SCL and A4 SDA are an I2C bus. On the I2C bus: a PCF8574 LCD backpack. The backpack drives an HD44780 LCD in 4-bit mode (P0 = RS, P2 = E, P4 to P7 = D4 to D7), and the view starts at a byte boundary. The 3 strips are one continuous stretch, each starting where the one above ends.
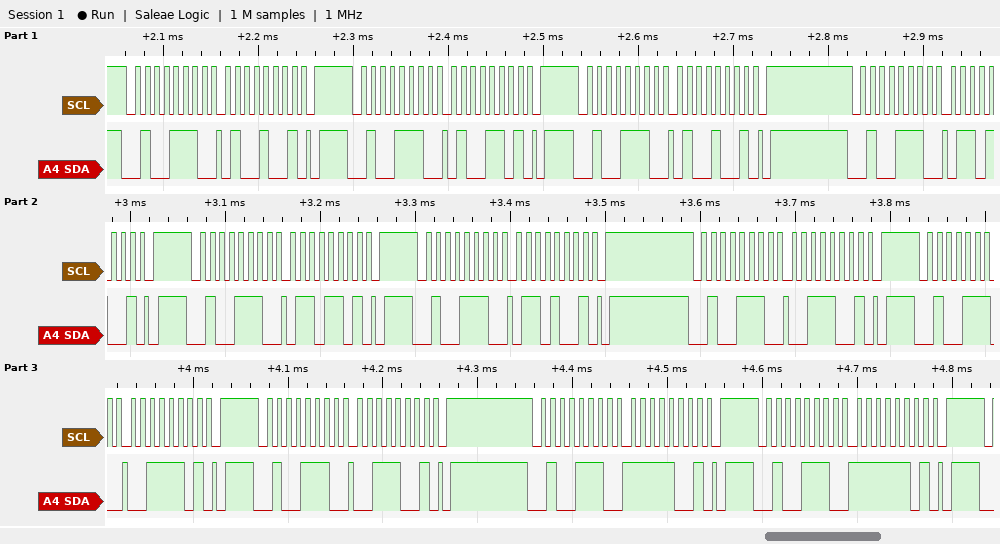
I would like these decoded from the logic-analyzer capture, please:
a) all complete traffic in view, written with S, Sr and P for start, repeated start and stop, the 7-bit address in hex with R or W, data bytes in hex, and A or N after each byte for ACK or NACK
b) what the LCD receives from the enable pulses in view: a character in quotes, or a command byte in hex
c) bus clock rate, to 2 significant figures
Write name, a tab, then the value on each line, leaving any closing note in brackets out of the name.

all complete traffic in view, written with S, Sr and P for start, repeated start and stop, the 7-bit address in hex with R or W, data bytes in hex, and A or N after each byte for ACK or NACK	S 27W A 49 A P S 27W A 4D A P S 27W A 49 A P S 27W A 69 A P S 27W A 6D A P S 27W A 69 A P S 27W A 39 A P S 27W A 3D A P S 27W A 39 A P S 27W A F9 A P S 27W A FD A P
what the LCD receives from the enable pulses in view: a character in quotes, or a command byte in hex	'F'
bus clock rate, to 2 significant figures	100 kHz
